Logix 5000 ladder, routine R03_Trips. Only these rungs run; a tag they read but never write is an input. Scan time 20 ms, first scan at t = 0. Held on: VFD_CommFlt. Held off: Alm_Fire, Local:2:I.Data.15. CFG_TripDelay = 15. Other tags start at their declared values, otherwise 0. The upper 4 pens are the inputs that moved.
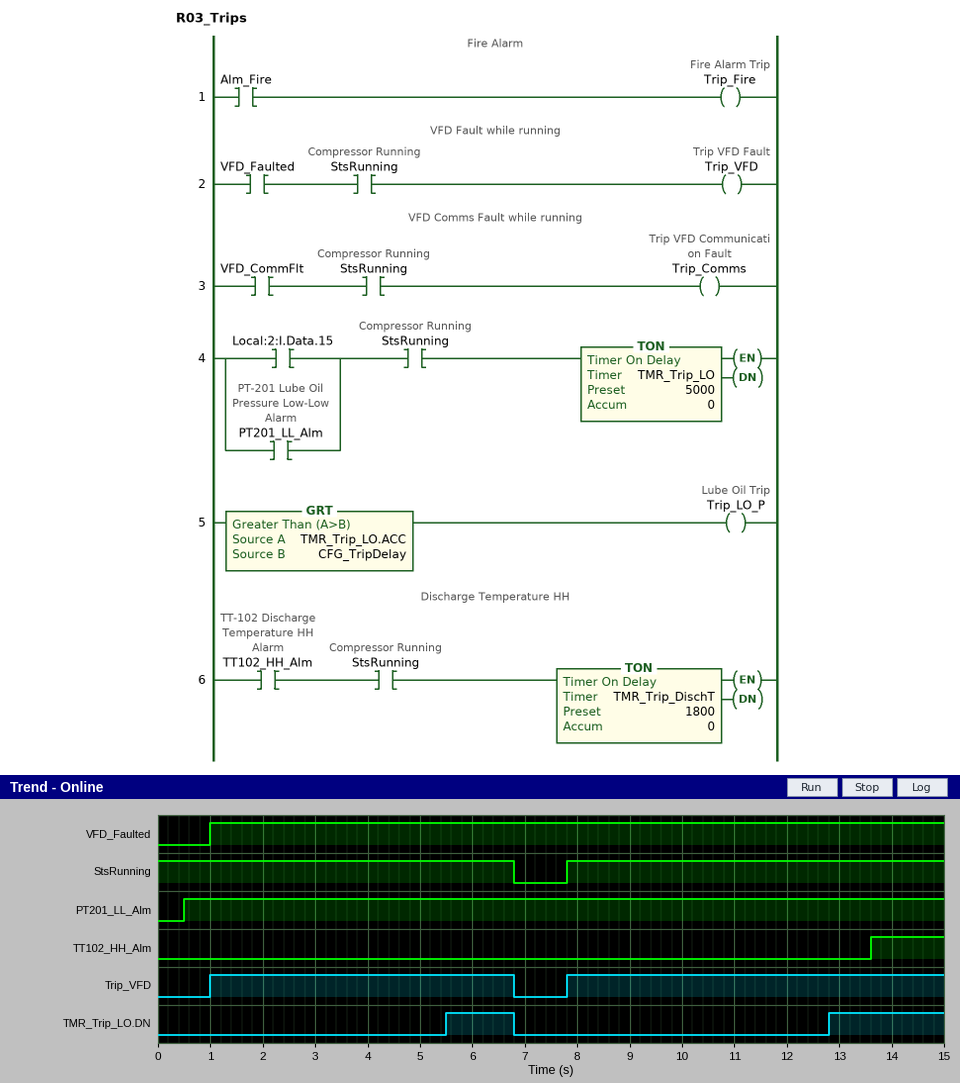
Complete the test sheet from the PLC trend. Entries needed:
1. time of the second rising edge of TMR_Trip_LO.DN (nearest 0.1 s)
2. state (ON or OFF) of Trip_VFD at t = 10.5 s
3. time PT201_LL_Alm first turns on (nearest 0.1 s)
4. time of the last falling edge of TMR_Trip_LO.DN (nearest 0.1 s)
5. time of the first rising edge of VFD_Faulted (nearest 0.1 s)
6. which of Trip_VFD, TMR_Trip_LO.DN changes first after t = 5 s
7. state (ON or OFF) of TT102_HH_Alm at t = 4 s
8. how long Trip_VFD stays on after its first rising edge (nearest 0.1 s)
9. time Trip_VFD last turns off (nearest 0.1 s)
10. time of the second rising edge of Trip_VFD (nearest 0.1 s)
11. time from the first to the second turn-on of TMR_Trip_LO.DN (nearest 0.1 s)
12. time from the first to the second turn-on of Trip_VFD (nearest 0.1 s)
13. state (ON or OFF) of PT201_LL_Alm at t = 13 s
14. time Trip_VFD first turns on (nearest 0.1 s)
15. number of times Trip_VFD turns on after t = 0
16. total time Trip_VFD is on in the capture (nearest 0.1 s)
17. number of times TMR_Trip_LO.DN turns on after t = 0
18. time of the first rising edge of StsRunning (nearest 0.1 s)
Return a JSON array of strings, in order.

["12.8 s", "ON", "0.5 s", "6.8 s", "1.0 s", "TMR_Trip_LO.DN", "OFF", "5.8 s", "6.8 s", "7.8 s", "7.3 s", "6.8 s", "ON", "1.0 s", "2", "13.0 s", "2", "7.8 s"]
